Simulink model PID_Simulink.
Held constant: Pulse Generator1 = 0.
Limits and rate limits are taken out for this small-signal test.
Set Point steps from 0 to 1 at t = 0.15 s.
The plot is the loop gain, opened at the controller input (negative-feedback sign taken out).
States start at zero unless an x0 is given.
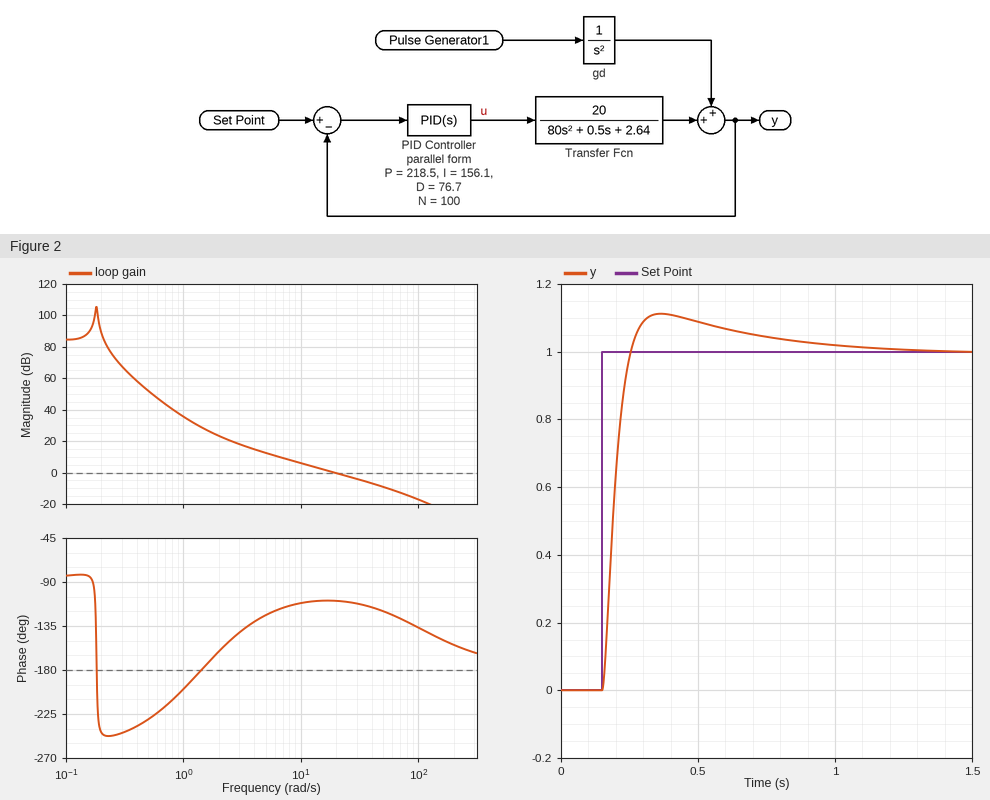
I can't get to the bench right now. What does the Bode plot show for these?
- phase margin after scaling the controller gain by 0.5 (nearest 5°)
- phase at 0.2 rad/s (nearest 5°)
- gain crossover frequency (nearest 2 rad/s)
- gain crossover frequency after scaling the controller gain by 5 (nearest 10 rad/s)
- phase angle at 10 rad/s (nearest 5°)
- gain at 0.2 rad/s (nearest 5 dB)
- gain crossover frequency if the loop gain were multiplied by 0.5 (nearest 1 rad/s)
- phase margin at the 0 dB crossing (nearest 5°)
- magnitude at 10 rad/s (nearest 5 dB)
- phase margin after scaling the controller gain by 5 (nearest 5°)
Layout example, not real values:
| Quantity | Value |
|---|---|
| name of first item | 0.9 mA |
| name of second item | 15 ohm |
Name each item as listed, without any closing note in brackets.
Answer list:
| Quantity | Value |
|---|---|
| phase margin after scaling the controller gain by 0.5 | 70° |
| phase at 0.2 rad/s | -245° |
| gain crossover frequency | 20 rad/s |
| gain crossover frequency after scaling the controller gain by 5 | 80 rad/s |
| phase angle at 10 rad/s | -110° |
| gain at 0.2 rad/s | 90 dB |
| gain crossover frequency if the loop gain were multiplied by 0.5 | 10 rad/s |
| phase margin at the 0 dB crossing | 70° |
| magnitude at 10 rad/s | 5 dB |
| phase margin after scaling the controller gain by 5 | 50° |
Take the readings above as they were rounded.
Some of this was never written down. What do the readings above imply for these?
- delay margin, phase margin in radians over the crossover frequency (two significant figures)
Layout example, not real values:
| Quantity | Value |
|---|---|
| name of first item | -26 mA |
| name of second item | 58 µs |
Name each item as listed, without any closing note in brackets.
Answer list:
| Quantity | Value |
|---|---|
| delay margin, phase margin in radians over the crossover frequency | 0.061 s |
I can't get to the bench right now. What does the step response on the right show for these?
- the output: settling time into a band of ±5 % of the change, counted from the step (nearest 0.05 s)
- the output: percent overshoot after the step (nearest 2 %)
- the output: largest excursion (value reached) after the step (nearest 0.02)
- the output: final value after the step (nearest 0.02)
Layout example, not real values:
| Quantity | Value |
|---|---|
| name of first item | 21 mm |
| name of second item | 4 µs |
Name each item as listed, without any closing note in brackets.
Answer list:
| Quantity | Value |
|---|---|
| the output: settling time into a band of ±5 % of the change, counted from the step | 0.55 s |
| the output: percent overshoot after the step | 12 % |
| the output: largest excursion (value reached) after the step | 1.12 |
| the output: final value after the step | 1.00 |
